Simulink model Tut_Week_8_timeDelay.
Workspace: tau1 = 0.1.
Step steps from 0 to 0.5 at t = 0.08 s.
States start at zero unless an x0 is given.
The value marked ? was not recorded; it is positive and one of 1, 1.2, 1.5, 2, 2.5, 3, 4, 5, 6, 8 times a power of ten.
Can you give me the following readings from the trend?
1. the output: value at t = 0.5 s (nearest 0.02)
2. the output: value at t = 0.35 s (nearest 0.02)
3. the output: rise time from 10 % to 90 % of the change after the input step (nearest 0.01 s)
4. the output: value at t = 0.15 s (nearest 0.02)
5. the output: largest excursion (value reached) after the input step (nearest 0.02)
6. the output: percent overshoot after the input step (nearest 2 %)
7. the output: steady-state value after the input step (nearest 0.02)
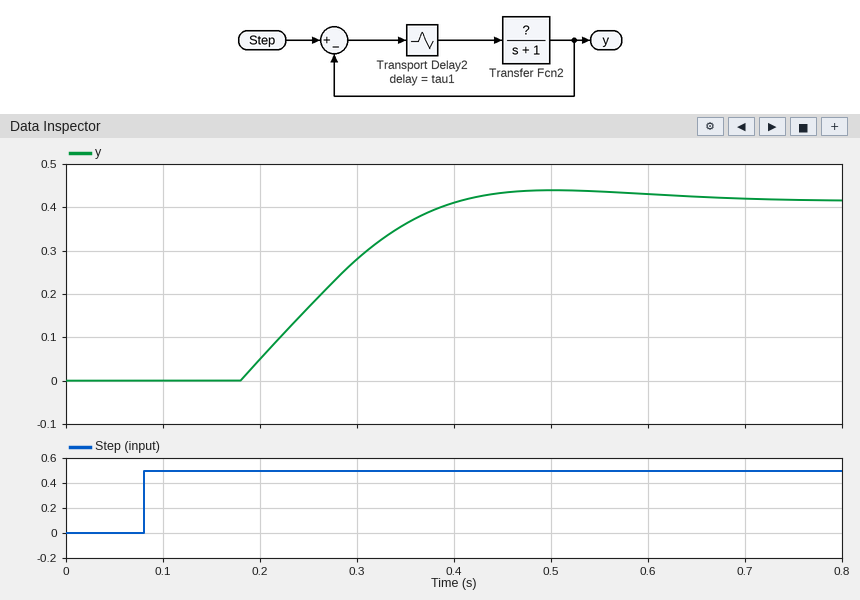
0.44
0.36
0.16 s
0.00
0.44
6 %
0.42
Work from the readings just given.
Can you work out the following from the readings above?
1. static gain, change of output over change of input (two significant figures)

0.84
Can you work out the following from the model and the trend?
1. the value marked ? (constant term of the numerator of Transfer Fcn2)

5
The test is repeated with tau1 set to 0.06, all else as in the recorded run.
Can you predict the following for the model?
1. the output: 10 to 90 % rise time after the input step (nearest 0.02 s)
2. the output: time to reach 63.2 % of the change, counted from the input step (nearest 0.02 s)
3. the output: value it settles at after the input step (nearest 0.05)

0.24 s
0.18 s
0.40
